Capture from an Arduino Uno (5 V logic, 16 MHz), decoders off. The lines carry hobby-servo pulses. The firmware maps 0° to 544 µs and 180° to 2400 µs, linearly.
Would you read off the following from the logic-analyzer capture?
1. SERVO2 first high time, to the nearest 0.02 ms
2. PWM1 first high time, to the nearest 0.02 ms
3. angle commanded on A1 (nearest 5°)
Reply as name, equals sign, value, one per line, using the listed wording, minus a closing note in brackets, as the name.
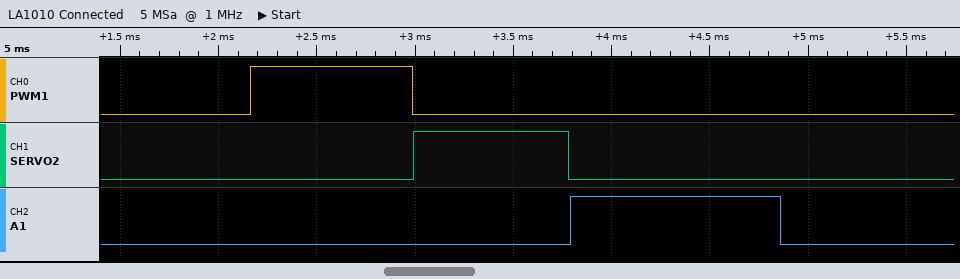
SERVO2 first high time, to the nearest 0.02 ms = 0.78 ms
PWM1 first high time, to the nearest 0.02 ms = 0.82 ms
angle commanded on A1 = 50°
